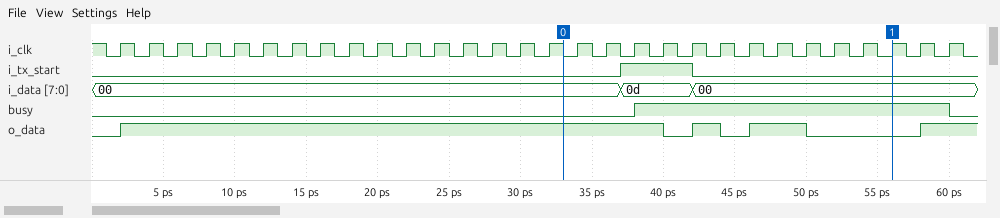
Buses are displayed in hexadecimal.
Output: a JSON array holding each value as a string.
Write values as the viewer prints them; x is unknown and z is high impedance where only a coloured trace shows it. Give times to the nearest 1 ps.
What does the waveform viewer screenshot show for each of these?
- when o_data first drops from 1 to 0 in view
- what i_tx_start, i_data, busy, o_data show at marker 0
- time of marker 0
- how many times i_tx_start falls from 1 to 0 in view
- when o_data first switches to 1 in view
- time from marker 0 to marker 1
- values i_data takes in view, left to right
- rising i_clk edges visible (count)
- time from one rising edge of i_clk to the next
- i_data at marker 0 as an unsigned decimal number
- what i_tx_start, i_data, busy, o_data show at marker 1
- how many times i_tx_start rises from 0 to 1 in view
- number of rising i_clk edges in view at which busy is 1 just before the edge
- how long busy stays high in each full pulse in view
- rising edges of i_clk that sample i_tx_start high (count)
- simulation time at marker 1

["40 ps", "i_tx_start=0, i_data=00, busy=0, o_data=1", "33 ps", "1", "2 ps", "23 ps", "00, 0d, 00", "30", "2 ps", "0", "i_tx_start=0, i_data=00, busy=1, o_data=0", "1", "11", "22 ps", "3", "56 ps"]
